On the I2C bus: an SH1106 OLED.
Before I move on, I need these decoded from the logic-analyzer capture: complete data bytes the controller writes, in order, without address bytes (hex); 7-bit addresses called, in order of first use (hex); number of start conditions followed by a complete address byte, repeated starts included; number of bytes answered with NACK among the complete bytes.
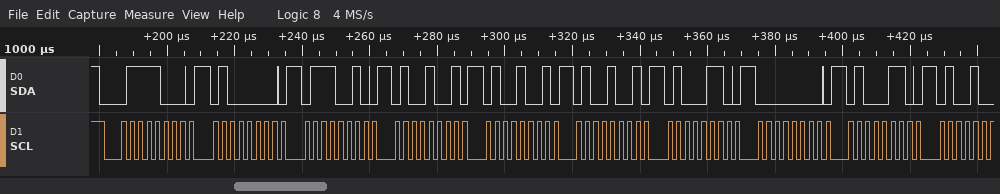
40 72 49 49 49 46 00 46
0x3C
1
0
